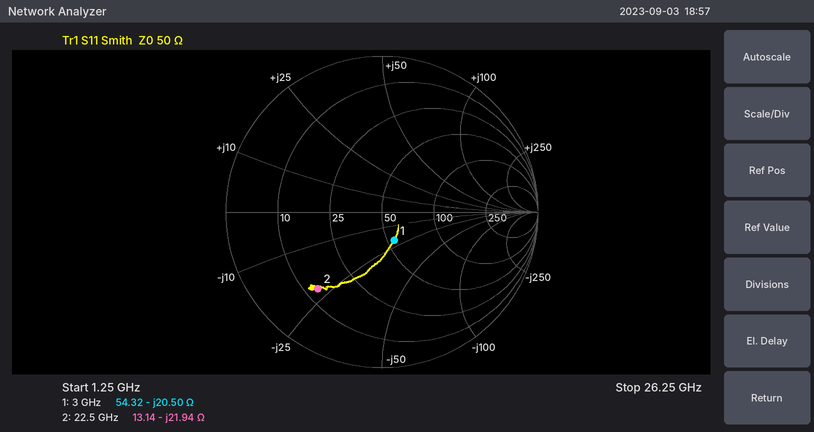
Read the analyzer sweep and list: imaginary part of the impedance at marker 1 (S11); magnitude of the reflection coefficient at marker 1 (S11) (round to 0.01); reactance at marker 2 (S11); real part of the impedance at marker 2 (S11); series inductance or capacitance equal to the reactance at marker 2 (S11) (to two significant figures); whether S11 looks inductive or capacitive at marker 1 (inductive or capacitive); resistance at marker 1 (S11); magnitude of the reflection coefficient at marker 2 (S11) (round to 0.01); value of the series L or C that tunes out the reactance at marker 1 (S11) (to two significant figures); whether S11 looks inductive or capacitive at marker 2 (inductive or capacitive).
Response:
-20.50 Ω
0.20
-21.94 Ω
13.14 Ω
320 fF
capacitive
54.32 Ω
0.64
1.1 nH
capacitive
